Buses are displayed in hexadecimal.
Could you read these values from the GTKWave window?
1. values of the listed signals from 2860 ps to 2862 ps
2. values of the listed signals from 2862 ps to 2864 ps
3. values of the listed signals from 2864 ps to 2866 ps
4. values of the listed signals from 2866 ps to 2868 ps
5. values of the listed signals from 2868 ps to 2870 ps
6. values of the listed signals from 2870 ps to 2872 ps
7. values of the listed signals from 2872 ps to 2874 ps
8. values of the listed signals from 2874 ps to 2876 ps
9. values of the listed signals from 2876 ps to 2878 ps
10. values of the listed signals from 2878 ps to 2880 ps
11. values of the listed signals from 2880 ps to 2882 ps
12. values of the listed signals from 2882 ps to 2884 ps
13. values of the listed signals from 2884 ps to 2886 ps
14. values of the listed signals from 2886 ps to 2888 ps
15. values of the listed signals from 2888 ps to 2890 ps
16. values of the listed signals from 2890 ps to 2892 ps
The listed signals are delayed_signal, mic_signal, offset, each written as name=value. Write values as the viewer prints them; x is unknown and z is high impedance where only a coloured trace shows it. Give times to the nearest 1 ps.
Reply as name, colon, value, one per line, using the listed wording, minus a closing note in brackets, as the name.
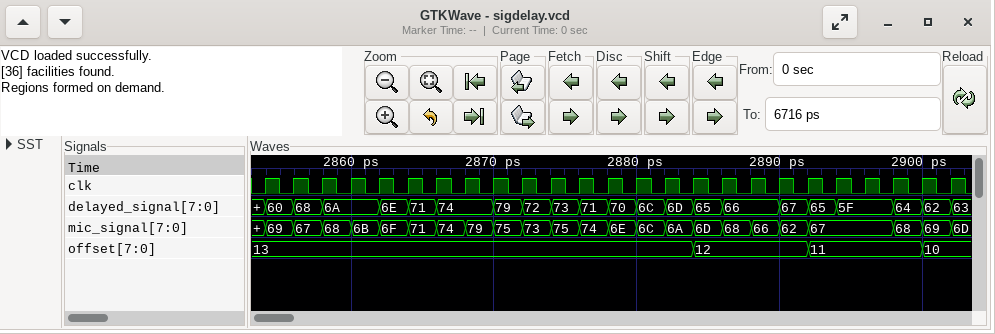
values of the listed signals from 2860 ps to 2862 ps: delayed_signal=6A, mic_signal=6B, offset=13
values of the listed signals from 2862 ps to 2864 ps: delayed_signal=6E, mic_signal=6F, offset=13
values of the listed signals from 2864 ps to 2866 ps: delayed_signal=71, mic_signal=71, offset=13
values of the listed signals from 2866 ps to 2868 ps: delayed_signal=74, mic_signal=74, offset=13
values of the listed signals from 2868 ps to 2870 ps: delayed_signal=74, mic_signal=79, offset=13
values of the listed signals from 2870 ps to 2872 ps: delayed_signal=79, mic_signal=75, offset=13
values of the listed signals from 2872 ps to 2874 ps: delayed_signal=72, mic_signal=73, offset=13
values of the listed signals from 2874 ps to 2876 ps: delayed_signal=73, mic_signal=75, offset=13
values of the listed signals from 2876 ps to 2878 ps: delayed_signal=71, mic_signal=74, offset=13
values of the listed signals from 2878 ps to 2880 ps: delayed_signal=70, mic_signal=6E, offset=13
values of the listed signals from 2880 ps to 2882 ps: delayed_signal=6C, mic_signal=6C, offset=13
values of the listed signals from 2882 ps to 2884 ps: delayed_signal=6D, mic_signal=6A, offset=13
values of the listed signals from 2884 ps to 2886 ps: delayed_signal=65, mic_signal=6D, offset=12
values of the listed signals from 2886 ps to 2888 ps: delayed_signal=66, mic_signal=68, offset=12
values of the listed signals from 2888 ps to 2890 ps: delayed_signal=66, mic_signal=66, offset=12
values of the listed signals from 2890 ps to 2892 ps: delayed_signal=67, mic_signal=62, offset=12
